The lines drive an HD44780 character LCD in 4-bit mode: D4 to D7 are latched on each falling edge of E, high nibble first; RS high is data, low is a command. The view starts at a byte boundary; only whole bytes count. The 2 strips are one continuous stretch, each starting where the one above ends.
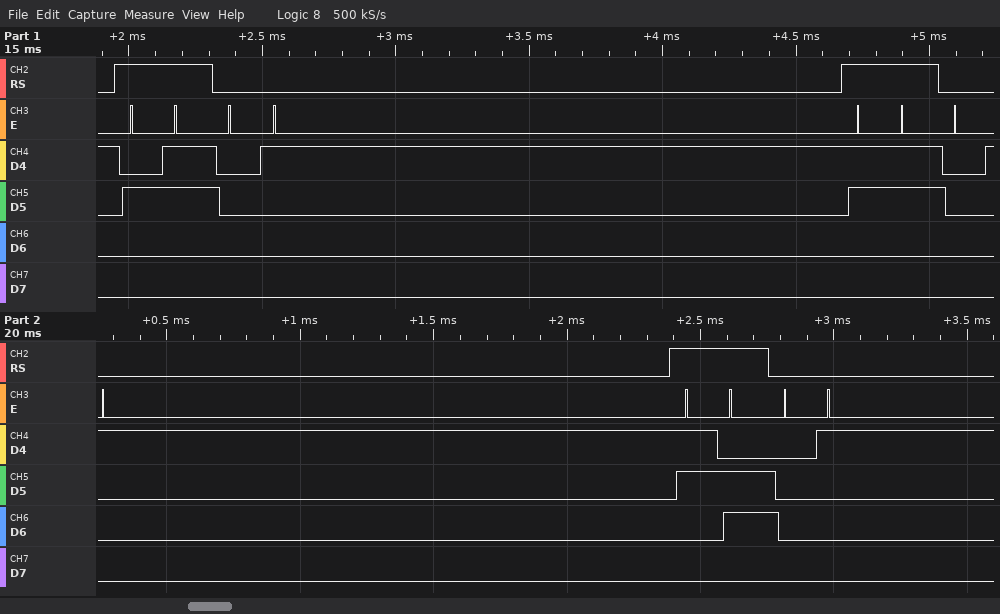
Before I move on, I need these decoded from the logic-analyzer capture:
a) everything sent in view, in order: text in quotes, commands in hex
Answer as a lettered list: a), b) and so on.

a) "#" 0x01 "3" 0x01 "6" 0x01
